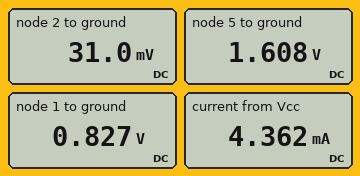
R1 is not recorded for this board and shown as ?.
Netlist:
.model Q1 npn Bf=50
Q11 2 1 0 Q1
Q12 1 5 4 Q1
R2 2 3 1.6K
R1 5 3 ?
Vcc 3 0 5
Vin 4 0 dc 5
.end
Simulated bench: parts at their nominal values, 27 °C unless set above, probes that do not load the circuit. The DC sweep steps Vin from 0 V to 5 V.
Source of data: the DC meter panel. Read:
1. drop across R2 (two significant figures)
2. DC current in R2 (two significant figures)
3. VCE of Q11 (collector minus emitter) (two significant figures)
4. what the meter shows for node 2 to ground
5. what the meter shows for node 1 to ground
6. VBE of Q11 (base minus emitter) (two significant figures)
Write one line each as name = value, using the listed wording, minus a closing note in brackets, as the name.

drop across R2 = 5.0 V
DC current in R2 = 3.1 mA
VCE of Q11 (collector minus emitter) = 31 mV
what the meter shows for node 2 to ground = 31.0 mV
what the meter shows for node 1 to ground = 0.827 V
VBE of Q11 (base minus emitter) = 830 mV
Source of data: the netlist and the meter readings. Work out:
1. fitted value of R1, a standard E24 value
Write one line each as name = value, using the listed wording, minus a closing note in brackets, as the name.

fitted value of R1, a standard E24 value = 2.7 kΩ
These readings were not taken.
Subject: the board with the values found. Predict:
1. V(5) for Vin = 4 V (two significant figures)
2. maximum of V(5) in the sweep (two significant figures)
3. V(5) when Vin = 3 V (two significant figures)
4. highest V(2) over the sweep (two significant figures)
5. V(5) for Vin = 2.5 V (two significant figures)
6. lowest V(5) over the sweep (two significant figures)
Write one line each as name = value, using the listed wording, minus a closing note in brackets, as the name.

V(5) for Vin = 4 V = 1.6 V
maximum of V(5) in the sweep = 1.6 V
V(5) when Vin = 3 V = 1.6 V
highest V(2) over the sweep = 5.0 V
V(5) for Vin = 2.5 V = 1.6 V
lowest V(5) over the sweep = 800 mV
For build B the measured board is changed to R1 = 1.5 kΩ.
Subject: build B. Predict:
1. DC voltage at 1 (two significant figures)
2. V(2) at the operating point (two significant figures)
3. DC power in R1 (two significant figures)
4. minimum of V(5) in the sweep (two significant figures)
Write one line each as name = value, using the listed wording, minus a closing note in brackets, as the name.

DC voltage at 1 = 840 mV
V(2) at the operating point = 26 mV
DC power in R1 = 7.6 mW
minimum of V(5) in the sweep = 820 mV
